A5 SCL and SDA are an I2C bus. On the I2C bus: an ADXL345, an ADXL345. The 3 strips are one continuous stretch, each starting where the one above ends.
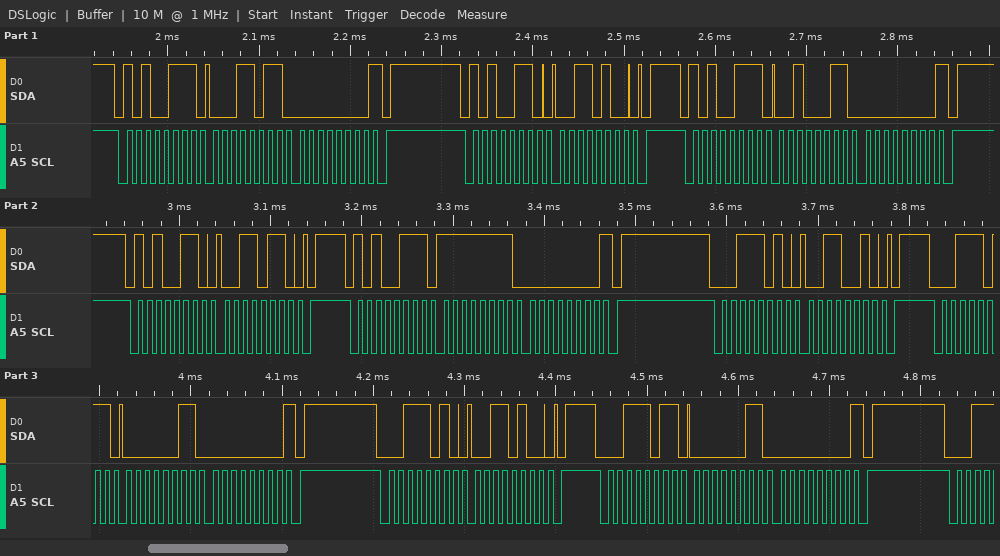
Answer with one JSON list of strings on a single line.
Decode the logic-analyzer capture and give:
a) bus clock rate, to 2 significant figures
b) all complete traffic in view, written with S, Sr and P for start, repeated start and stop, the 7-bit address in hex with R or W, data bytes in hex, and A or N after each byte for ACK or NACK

["100 kHz", "S 53R A 1B A 00 N P S 53W A 34 A P S 53R A 23 A 00 N P S 53W A 36 A P S 53R A FF A 00 N P S 1DW A 32 A P S 1DR A 03 A 00 N P S 1DW A 34 A P S 1DR A 03 A 00 N P"]
